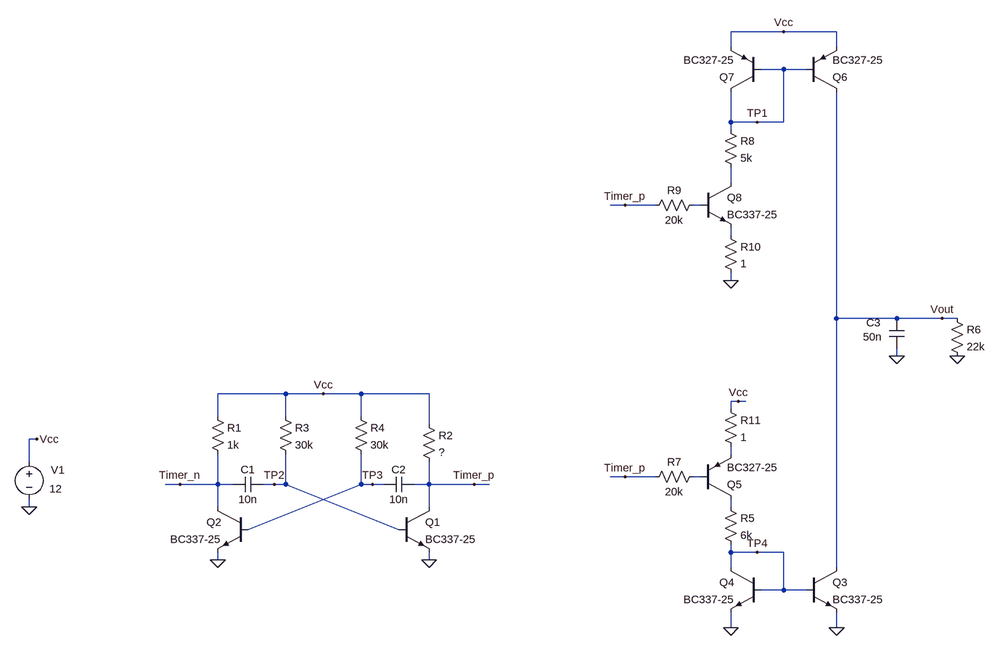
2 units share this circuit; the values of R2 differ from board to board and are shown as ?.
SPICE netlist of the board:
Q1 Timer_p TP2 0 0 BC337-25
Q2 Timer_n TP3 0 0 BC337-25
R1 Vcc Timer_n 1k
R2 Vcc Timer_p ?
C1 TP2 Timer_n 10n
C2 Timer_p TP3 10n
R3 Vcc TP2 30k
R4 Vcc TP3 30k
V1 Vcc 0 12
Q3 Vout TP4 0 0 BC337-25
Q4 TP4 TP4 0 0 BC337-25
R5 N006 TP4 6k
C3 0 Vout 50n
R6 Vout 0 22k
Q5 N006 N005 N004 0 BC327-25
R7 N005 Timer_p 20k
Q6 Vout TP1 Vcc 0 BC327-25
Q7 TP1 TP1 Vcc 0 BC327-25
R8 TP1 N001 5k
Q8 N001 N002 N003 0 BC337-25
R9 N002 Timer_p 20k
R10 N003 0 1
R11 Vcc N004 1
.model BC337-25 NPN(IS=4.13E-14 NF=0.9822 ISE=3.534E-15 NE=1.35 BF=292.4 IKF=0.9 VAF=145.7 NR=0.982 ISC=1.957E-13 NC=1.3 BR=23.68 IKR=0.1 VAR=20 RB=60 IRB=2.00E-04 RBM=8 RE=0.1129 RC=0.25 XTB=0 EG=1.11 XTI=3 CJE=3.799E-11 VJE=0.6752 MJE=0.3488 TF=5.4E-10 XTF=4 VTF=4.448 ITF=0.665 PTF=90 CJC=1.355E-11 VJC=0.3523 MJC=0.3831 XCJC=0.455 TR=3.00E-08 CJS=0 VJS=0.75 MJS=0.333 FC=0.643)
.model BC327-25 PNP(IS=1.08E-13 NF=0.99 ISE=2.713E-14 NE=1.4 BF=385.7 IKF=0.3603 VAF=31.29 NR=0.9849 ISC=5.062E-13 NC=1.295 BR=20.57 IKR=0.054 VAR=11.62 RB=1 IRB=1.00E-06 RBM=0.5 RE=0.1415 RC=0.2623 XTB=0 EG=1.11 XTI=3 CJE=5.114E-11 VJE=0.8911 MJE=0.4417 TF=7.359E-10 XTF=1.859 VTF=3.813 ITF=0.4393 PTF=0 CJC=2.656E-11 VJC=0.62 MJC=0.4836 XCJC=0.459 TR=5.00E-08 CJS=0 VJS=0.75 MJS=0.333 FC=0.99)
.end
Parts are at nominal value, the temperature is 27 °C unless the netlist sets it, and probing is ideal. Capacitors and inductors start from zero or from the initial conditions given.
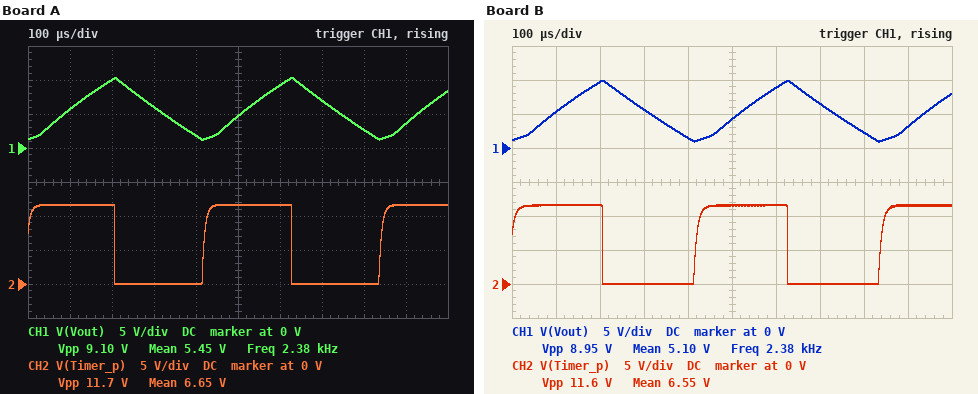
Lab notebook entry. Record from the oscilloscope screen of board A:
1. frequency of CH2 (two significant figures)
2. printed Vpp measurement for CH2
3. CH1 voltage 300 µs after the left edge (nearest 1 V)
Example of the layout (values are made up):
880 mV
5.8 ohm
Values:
2.4 kHz
11.7 V
6 V
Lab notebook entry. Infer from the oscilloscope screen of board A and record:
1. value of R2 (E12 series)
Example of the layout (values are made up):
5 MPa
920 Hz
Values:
680 Ω
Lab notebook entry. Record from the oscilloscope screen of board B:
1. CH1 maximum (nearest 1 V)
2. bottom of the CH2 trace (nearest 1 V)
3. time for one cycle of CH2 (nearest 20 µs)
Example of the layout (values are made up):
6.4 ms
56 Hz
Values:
10 V
0 V
420 µs
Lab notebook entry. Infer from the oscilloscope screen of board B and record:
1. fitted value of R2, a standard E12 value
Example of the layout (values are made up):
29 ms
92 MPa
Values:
820 Ω
